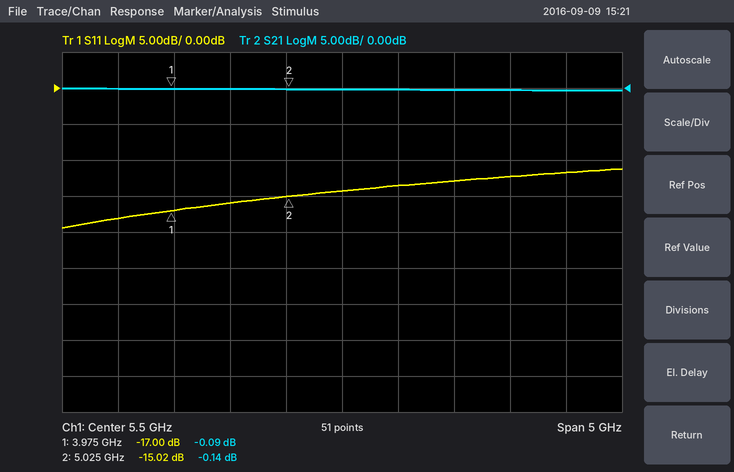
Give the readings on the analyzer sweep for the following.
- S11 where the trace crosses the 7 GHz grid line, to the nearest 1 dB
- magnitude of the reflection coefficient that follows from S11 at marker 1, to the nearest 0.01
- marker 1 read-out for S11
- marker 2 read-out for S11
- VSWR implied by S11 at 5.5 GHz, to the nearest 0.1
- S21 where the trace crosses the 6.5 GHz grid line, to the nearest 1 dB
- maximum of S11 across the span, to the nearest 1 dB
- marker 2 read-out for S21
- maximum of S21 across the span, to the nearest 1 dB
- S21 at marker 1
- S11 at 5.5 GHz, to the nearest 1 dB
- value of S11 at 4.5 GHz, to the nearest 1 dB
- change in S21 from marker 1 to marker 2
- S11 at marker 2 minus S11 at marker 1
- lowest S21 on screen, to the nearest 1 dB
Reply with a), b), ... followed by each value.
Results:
a) -12 dB
b) 0.14
c) -17.00 dB
d) -15.02 dB
e) 1.5
f) 0 dB
g) -11 dB
h) -0.14 dB
i) 0 dB
j) -0.09 dB
k) -14 dB
l) -16 dB
m) -0.05 dB
n) 1.98 dB
o) 0 dB
